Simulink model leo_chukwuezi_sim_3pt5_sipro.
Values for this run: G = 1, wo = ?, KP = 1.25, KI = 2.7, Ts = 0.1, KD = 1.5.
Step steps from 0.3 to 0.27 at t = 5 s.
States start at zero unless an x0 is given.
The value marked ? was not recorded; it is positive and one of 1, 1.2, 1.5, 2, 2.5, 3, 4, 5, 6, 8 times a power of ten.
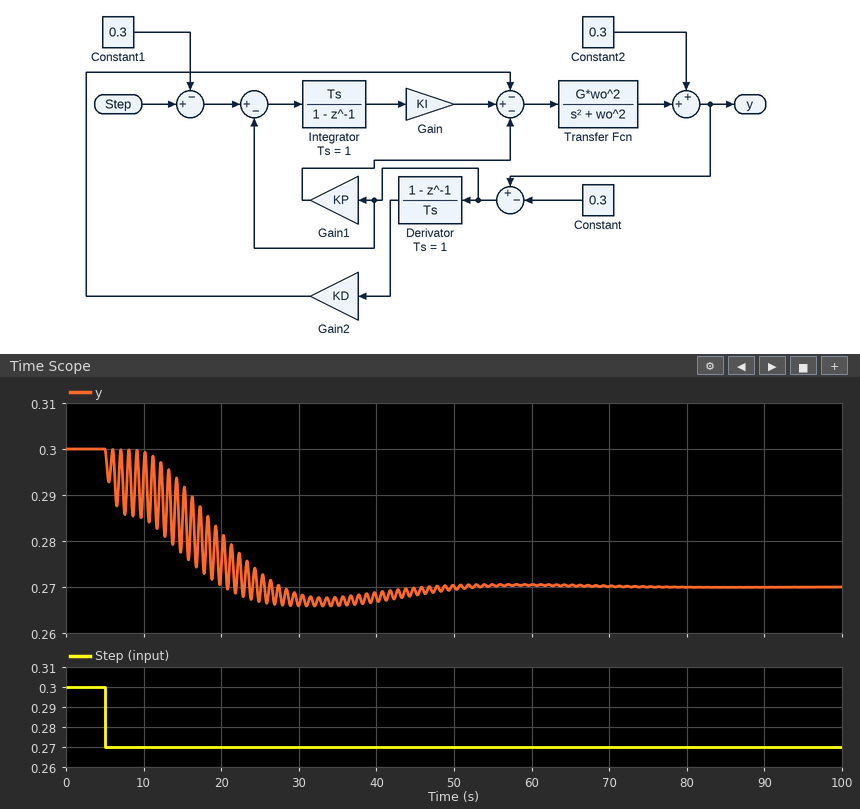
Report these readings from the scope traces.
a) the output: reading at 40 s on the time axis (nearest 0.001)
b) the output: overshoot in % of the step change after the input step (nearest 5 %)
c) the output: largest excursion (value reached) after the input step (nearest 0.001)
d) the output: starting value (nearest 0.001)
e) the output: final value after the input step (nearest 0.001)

0.268
15 %
0.266
0.300
0.270
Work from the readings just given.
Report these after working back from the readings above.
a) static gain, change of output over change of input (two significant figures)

1.0
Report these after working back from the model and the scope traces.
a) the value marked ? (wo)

4
